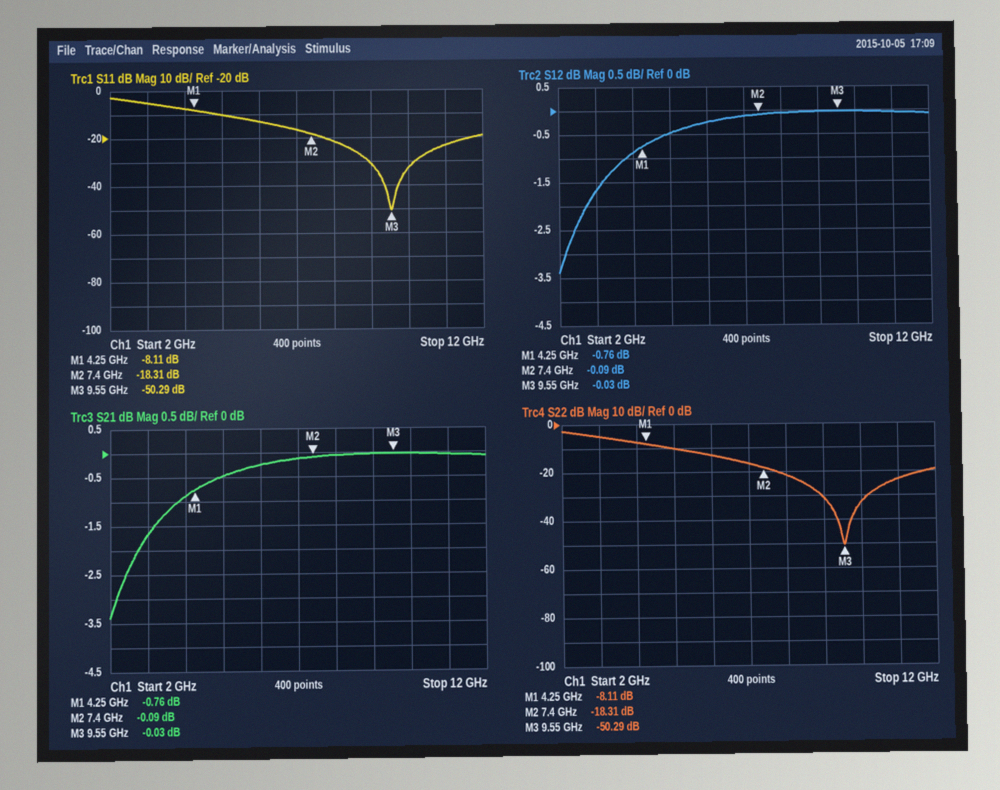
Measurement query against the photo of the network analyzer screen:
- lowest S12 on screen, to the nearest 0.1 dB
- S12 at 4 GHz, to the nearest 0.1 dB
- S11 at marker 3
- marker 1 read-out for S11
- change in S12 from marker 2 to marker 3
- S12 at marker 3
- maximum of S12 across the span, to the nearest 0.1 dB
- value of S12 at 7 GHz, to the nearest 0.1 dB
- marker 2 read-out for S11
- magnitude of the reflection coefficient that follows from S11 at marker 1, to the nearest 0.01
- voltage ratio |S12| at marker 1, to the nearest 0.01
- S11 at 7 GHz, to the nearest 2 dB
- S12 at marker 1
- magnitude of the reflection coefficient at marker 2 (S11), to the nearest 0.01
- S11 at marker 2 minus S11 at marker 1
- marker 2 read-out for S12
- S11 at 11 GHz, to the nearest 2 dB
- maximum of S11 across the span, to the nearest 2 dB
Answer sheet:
-3.4 dB
-0.9 dB
-50.29 dB
-8.11 dB
0.06 dB
-0.03 dB
0.0 dB
-0.1 dB
-18.31 dB
0.39
0.92
-16 dB
-0.76 dB
0.12
-10.20 dB
-0.09 dB
-24 dB
-2 dB
